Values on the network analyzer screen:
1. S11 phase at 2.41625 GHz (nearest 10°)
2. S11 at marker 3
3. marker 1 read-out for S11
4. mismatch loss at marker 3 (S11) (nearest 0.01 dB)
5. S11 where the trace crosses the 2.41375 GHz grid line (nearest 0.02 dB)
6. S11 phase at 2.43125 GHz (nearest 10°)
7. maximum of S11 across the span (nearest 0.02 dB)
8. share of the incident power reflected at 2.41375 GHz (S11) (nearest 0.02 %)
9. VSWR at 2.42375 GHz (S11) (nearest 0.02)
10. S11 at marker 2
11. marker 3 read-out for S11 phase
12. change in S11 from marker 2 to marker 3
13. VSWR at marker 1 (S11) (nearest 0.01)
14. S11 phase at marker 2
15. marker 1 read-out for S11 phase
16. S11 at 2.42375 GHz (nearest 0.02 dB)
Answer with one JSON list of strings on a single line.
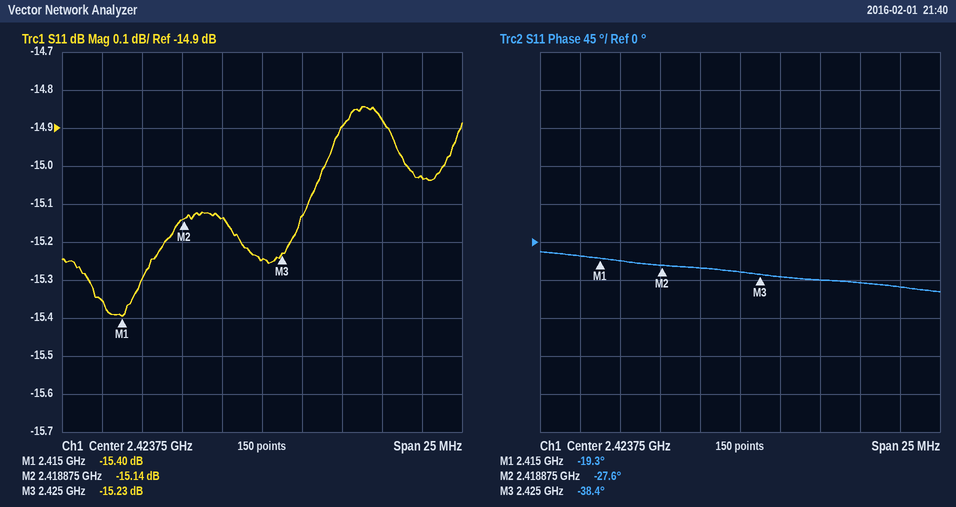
["-20°", "-15.23 dB", "-15.40 dB", "0.13 dB", "-15.36 dB", "-50°", "-14.84 dB", "2.92 %", "1.42", "-15.14 dB", "-38.4°", "-0.09 dB", "1.41", "-27.6°", "-19.3°", "-15.24 dB"]
